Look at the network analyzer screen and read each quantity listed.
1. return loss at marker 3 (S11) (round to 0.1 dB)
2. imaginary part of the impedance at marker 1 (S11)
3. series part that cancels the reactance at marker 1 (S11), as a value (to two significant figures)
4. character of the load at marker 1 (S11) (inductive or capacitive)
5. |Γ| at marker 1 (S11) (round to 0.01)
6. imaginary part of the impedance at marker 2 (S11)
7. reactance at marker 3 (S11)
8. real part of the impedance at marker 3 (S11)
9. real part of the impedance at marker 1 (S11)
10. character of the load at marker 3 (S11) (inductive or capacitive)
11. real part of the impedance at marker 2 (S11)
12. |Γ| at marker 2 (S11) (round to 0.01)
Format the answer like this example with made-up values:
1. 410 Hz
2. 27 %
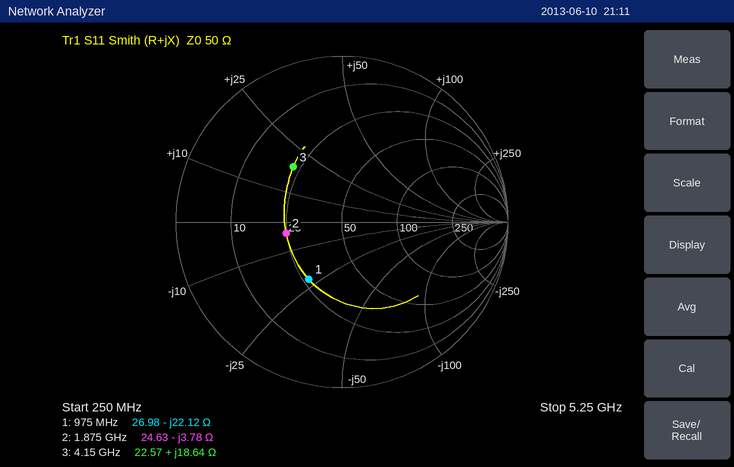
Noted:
1. 7.1 dB
2. -22.12 Ω
3. 3.6 nH
4. capacitive
5. 0.40
6. -3.78 Ω
7. +18.64 Ω
8. 22.57 Ω
9. 26.98 Ω
10. inductive
11. 24.63 Ω
12. 0.34
